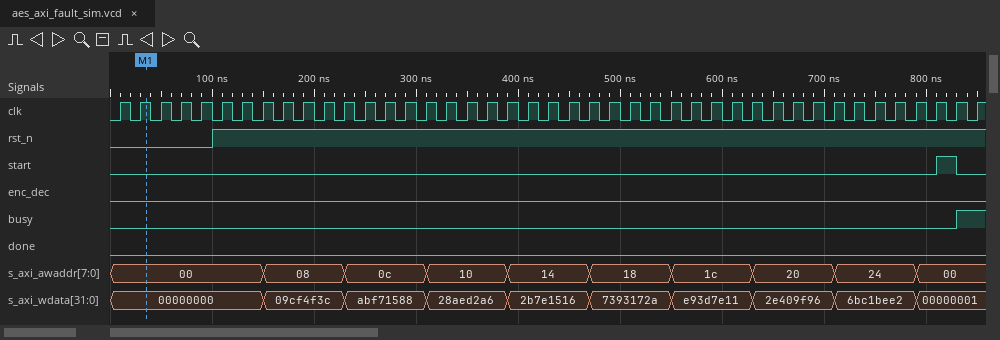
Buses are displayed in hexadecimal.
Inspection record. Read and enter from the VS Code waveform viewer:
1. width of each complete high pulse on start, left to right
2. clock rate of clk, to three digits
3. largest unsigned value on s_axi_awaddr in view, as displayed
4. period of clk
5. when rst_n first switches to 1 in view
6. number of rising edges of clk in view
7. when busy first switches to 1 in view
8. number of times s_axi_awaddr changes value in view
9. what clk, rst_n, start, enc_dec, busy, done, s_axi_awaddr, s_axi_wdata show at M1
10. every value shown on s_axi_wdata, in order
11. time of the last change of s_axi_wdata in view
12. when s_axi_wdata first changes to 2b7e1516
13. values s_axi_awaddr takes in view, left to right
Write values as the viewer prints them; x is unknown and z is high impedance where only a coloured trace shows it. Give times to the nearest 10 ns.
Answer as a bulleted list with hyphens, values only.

- 20 ns
- 50.0 MHz
- 24
- 20 ns
- 100 ns
- 43
- 830 ns
- 9
- clk=1, rst_n=0, start=0, enc_dec=0, busy=0, done=0, s_axi_awaddr=00, s_axi_wdata=00000000
- 00000000, 09cf4f3c, abf71588, 28aed2a6, 2b7e1516, 7393172a, e93d7e11, 2e409f96, 6bc1bee2, 00000001
- 790 ns
- 390 ns
- 00, 08, 0c, 10, 14, 18, 1c, 20, 24, 00
